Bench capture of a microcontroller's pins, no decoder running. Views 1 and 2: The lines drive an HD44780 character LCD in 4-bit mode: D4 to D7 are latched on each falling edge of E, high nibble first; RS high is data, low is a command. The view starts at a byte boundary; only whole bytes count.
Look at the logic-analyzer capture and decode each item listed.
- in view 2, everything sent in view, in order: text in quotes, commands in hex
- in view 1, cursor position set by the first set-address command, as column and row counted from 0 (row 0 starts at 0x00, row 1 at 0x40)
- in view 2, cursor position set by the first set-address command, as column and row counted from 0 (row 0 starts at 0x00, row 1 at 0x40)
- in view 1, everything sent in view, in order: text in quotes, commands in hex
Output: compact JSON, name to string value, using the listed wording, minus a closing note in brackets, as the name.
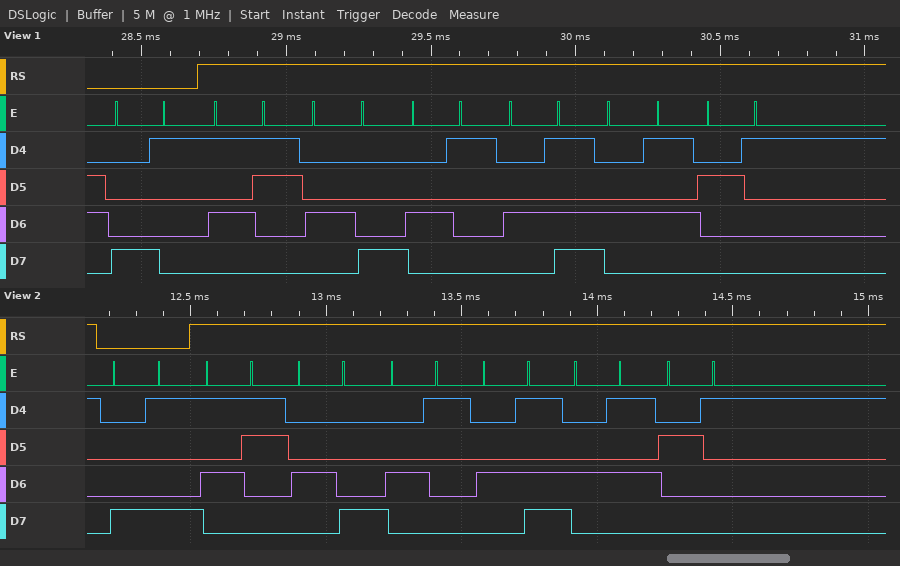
{"in view 2, everything sent in view, in order: text in quotes, commands in hex": "0x89 \"SHAME!\"", "in view 1, cursor position set by the first set-address command, as column and row counted from 0": "column 1, row 0", "in view 2, cursor position set by the first set-address command, as column and row counted from 0": "column 9, row 0", "in view 1, everything sent in view, in order: text in quotes, commands in hex": "0x81 \"SHAME!\""}
